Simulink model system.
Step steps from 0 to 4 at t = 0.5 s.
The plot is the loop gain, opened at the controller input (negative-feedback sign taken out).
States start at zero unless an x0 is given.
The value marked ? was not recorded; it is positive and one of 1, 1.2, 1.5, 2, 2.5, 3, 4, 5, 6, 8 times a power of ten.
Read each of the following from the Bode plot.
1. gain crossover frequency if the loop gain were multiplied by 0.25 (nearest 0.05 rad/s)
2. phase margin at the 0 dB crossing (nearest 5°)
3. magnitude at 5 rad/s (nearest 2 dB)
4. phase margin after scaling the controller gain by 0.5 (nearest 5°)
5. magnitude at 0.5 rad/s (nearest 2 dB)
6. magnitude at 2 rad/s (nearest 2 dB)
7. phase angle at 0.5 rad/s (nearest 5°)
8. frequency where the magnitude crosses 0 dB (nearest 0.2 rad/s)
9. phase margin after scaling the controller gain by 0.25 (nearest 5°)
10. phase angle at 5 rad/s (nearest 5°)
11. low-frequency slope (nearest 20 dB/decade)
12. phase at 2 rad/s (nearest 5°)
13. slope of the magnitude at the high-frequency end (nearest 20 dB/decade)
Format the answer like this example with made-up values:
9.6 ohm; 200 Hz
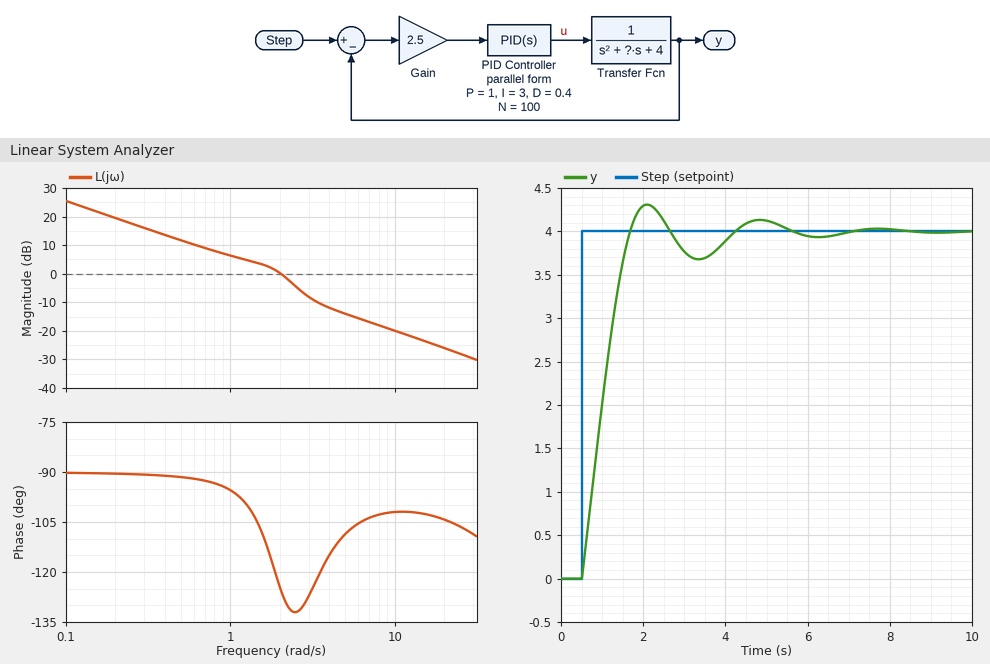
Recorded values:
0.50 rad/s; 55°; -14 dB; 85°; 12 dB; 0 dB; -90°; 2.0 rad/s; 90°; -110°; -20 dB/decade; -125°; -20 dB/decade
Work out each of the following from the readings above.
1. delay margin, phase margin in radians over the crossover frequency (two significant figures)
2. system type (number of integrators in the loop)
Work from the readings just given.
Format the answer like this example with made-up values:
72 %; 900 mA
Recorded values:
0.48 s; 1
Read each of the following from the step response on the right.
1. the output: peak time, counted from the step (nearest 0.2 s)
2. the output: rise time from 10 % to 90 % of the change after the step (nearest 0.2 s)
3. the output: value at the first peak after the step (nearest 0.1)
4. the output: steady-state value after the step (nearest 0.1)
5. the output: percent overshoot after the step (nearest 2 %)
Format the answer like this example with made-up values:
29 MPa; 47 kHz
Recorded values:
1.6 s; 0.8 s; 4.3; 4.0; 8 %
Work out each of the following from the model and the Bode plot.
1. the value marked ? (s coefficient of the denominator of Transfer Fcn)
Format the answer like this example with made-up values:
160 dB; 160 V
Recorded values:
1.5
